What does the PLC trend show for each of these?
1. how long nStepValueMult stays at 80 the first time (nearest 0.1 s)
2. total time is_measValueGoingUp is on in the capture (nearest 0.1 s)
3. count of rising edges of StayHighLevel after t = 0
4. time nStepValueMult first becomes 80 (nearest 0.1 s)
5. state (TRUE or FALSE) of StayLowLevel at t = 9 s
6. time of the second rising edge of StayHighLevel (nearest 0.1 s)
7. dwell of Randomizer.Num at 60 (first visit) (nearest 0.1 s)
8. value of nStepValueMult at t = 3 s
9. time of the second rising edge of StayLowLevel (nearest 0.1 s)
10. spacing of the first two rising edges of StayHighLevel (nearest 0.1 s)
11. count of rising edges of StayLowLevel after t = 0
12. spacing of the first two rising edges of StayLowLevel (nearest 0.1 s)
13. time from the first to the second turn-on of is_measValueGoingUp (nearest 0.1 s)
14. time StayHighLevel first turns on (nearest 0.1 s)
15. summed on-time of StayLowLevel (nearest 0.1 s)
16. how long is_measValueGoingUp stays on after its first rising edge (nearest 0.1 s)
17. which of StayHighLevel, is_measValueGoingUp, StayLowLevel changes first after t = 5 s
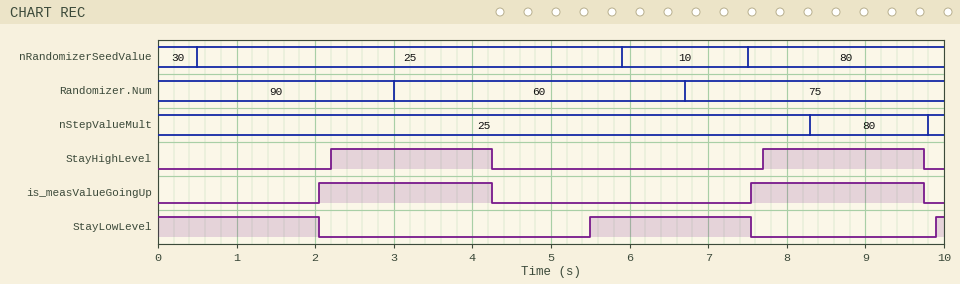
1.5 s
4.4 s
2
8.3 s
FALSE
7.7 s
3.7 s
25
9.9 s
5.5 s
2
4.4 s
5.5 s
2.2 s
4.2 s
2.2 s
StayLowLevel
